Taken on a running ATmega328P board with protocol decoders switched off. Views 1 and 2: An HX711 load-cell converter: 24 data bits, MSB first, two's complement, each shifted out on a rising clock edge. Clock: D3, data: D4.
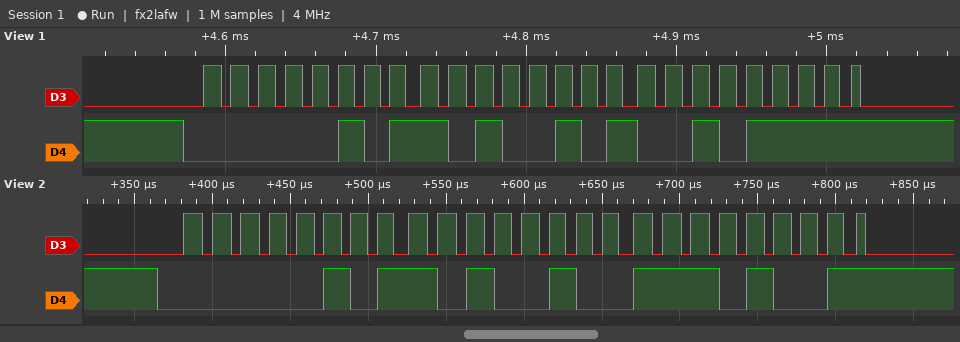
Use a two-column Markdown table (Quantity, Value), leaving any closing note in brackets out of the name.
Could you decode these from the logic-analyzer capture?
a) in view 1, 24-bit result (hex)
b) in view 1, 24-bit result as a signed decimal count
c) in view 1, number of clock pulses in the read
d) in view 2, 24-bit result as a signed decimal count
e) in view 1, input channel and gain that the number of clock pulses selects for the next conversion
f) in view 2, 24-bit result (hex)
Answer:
| Quantity | Value |
|---|---|
| in view 1, 24-bit result | 0x05A52F |
| in view 1, 24-bit result as a signed decimal count | 369967 |
| in view 1, number of clock pulses in the read | 25 |
| in view 2, 24-bit result as a signed decimal count | 369897 |
| in view 1, input channel and gain that the number of clock pulses selects for the next conversion | channel A, gain 128 |
| in view 2, 24-bit result | 0x05A4E9 |
